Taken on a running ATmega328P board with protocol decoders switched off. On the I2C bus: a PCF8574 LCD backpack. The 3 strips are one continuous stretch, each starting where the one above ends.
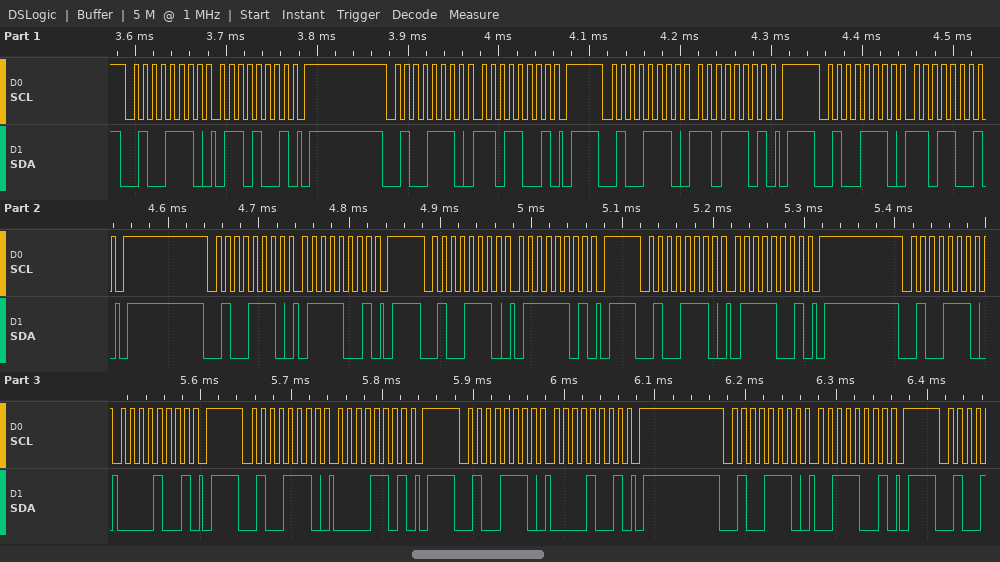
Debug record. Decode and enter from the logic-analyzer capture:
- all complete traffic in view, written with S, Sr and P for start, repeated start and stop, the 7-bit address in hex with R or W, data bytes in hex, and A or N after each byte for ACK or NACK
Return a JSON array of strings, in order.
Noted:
["S 27W A 69 A P S 27W A D9 A P S 27W A DD A P S 27W A D9 A P S 27W A 79 A P S 27W A 7D A P S 27W A 79 A P S 27W A 09 A P S 27W A 0D A P S 27W A 09 A P S 27W A 39 A P"]
